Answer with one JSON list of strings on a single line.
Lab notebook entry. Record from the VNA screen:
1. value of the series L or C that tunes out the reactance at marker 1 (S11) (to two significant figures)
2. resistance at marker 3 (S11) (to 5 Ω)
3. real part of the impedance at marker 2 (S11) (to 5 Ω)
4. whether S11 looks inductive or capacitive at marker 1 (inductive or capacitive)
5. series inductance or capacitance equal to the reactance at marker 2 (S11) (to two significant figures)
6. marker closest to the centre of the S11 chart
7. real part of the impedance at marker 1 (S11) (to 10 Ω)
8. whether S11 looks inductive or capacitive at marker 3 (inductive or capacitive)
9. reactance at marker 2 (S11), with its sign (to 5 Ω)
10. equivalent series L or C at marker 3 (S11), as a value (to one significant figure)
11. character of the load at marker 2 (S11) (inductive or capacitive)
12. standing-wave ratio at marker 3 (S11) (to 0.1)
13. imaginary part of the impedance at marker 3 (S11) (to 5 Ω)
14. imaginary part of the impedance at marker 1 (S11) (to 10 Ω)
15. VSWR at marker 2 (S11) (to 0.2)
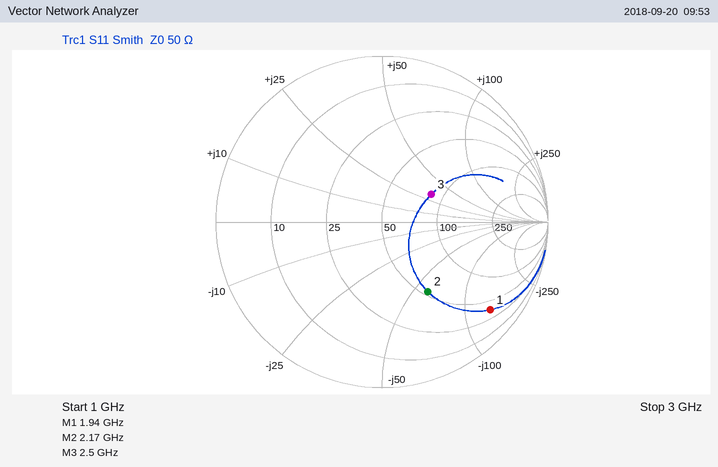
["11 nH", "85 Ω", "55 Ω", "capacitive", "1.2 pF", "marker 3", "40 Ω", "inductive", "-60 Ω", "2 nH", "capacitive", "2.0", "+30 Ω", "-130 Ω", "3.0"]
